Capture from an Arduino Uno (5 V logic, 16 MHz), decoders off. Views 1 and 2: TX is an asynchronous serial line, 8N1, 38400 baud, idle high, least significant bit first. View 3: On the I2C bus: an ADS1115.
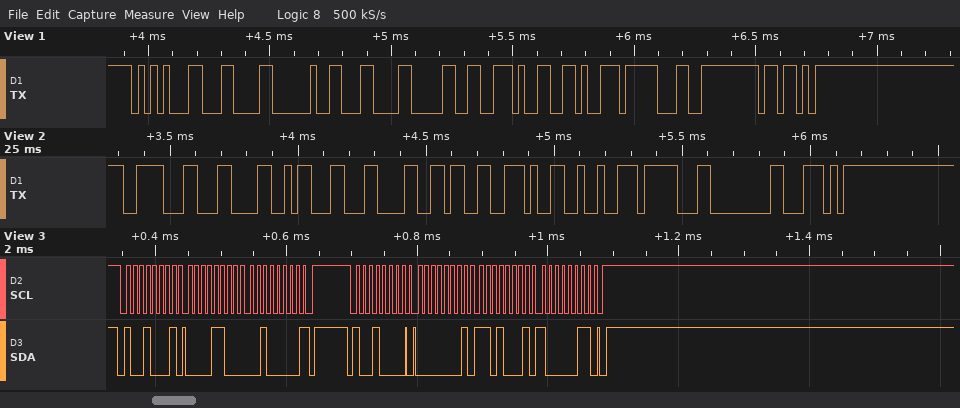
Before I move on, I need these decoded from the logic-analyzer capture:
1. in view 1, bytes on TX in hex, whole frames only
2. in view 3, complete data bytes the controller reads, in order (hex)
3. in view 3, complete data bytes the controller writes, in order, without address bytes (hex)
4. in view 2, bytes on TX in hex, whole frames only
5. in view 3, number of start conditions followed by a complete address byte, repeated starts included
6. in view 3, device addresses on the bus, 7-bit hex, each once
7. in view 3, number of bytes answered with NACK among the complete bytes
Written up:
15 0C 20 0C 30 2E 96 1F FE 5B
0C 20
01 D1 83
1E 0C 1A 0C 36 2E 92 1F 00 5C
2
0x48
1
